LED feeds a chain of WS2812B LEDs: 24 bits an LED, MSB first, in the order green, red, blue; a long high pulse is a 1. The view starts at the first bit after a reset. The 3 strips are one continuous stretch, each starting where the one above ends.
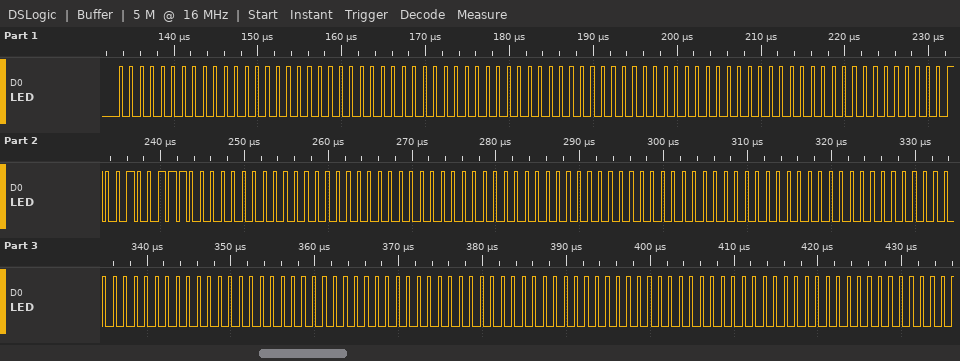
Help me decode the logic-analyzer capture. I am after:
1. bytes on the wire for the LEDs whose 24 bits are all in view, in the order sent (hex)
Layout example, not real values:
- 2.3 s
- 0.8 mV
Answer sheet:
- 00 00 00 00 00 00 00 00 00 01 27 00 00 00 00 00 00 00 00 00 00 00 00 00 00 00 00 00 00 00
